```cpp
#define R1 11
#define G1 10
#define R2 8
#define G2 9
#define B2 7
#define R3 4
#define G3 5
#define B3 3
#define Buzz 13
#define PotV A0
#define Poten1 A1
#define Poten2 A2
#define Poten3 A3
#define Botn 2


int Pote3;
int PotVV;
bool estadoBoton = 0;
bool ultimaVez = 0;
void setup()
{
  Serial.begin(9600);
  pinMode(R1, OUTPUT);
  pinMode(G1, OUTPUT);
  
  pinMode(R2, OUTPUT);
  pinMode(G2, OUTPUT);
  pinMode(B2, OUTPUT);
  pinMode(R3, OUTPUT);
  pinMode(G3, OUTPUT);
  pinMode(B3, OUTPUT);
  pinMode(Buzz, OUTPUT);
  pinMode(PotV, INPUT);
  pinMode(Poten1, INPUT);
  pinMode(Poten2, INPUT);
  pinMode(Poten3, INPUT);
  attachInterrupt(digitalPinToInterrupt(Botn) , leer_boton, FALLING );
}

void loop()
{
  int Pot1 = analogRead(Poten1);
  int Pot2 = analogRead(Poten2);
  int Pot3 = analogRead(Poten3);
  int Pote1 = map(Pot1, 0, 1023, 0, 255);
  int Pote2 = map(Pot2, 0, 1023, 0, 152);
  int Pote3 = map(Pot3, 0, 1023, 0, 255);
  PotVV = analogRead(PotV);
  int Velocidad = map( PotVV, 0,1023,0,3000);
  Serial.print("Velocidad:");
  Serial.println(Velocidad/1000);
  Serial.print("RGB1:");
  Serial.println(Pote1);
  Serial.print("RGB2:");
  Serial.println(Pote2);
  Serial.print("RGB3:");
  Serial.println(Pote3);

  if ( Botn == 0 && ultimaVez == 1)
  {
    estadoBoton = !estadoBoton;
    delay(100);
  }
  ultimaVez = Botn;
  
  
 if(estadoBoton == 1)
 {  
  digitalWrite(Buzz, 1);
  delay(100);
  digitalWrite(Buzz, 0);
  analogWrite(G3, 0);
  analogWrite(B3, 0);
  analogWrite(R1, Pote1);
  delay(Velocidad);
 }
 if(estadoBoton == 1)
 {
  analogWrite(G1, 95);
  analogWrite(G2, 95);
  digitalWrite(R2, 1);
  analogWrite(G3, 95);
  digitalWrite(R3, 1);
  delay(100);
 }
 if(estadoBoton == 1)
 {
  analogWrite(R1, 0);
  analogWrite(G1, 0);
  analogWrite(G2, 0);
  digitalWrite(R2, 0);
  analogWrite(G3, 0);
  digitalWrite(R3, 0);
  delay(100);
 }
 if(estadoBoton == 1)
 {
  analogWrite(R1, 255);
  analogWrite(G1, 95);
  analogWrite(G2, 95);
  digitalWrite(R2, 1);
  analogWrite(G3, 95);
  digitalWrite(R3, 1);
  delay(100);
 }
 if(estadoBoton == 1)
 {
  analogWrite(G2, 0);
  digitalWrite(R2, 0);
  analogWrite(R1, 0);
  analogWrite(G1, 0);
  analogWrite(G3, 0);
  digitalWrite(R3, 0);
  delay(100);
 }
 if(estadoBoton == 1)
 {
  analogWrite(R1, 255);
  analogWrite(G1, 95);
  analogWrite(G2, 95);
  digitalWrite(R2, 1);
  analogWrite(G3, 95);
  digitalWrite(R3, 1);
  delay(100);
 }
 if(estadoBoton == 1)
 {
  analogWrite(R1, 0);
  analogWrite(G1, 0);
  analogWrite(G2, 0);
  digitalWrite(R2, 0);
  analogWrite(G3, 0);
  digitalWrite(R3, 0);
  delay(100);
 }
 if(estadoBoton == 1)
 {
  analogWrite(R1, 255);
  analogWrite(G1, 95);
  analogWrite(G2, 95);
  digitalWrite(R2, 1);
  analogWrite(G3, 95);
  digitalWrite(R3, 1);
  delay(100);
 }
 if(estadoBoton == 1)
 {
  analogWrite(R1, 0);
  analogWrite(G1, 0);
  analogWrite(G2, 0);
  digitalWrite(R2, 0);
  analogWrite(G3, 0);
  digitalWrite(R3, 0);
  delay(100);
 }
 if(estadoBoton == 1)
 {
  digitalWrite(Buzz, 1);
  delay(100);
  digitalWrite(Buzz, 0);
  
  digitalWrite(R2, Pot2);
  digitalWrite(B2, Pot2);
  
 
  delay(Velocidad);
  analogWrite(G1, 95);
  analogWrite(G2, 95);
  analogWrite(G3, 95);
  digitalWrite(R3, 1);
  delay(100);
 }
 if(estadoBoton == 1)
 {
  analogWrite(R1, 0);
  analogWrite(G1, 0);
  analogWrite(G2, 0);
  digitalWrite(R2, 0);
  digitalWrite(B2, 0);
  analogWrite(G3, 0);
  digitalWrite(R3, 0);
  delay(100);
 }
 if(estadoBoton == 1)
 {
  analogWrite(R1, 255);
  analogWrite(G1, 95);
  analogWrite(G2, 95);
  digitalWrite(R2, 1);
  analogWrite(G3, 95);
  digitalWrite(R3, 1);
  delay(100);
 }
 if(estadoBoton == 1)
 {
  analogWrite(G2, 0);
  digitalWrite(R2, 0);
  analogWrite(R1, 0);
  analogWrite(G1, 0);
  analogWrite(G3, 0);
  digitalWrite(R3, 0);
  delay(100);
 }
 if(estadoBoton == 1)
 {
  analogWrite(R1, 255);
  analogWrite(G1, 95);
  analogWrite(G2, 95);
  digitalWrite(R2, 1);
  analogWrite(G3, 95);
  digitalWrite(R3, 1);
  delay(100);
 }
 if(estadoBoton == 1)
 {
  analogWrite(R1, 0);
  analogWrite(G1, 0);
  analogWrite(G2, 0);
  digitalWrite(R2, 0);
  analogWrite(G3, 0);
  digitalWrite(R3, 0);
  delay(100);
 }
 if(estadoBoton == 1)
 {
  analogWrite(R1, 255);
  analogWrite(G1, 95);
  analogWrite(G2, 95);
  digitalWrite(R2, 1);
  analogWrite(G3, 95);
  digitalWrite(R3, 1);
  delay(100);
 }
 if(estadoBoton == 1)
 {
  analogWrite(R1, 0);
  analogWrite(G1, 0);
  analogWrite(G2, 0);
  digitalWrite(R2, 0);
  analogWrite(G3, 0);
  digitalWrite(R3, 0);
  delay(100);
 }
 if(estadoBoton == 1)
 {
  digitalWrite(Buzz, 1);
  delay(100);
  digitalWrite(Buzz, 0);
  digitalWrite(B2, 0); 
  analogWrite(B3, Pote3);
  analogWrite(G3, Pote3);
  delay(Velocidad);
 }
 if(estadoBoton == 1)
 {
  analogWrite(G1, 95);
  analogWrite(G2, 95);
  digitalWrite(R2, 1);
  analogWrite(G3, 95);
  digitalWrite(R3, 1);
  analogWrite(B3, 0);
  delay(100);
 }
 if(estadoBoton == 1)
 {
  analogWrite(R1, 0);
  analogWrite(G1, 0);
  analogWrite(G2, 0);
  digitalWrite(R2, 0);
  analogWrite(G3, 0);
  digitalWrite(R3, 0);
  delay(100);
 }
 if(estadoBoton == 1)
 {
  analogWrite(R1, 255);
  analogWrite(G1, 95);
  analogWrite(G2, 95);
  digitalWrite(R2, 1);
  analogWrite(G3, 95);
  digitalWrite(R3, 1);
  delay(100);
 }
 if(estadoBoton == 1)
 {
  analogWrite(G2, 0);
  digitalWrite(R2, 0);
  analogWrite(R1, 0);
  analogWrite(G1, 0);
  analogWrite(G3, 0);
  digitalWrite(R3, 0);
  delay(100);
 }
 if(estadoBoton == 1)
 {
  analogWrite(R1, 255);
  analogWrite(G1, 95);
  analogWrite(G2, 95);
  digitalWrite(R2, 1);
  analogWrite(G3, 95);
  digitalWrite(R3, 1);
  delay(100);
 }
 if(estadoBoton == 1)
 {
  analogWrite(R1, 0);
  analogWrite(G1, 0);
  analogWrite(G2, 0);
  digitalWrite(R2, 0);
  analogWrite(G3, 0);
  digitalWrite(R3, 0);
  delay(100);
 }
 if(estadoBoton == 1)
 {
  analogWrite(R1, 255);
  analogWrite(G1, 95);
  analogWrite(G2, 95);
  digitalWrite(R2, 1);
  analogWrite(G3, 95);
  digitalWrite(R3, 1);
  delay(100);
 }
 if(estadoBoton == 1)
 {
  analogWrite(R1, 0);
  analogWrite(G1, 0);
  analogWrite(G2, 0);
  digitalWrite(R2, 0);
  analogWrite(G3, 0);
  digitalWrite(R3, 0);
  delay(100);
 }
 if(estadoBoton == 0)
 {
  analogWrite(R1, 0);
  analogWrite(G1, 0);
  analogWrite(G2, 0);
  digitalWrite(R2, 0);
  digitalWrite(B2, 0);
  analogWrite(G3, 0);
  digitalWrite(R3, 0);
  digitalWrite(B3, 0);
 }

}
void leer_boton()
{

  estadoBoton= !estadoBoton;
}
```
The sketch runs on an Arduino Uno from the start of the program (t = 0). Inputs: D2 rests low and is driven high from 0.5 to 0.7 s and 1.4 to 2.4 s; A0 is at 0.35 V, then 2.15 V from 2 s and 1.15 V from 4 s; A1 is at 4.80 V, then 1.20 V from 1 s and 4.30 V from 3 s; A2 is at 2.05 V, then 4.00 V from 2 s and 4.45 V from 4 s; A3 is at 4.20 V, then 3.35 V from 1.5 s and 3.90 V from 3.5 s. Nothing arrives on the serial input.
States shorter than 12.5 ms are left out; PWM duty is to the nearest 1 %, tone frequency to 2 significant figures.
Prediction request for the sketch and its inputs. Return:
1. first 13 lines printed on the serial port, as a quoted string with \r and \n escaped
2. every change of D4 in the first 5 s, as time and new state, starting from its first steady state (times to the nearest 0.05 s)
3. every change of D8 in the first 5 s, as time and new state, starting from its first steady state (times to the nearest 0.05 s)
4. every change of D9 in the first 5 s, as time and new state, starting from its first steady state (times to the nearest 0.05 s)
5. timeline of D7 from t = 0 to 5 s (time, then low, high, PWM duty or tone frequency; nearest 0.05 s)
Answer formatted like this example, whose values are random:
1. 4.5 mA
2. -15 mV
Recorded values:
1. "Velocidad:0\r\nRGB1:245\r\nRGB2:62\r\nRGB3:214\r\nVelocidad:0\r\nRGB1:245\r\nRGB2:62\r\nRGB3:214\r\nVelocidad:0\r\nRGB1:245\r\nRGB2:62\r\nRGB3:214\r\nVelocidad:0\r\n"
2. 0 s low; 1.05 s high; 1.15 s low; 1.25 s high; 1.35 s low; 1.45 s high; 1.55 s low; 1.65 s high; 1.75 s low; 2.15 s high; 2.25 s low; 2.35 s high; 2.45 s low
3. 0 s low; 1.05 s high; 1.15 s low; 1.25 s high; 1.35 s low; 1.45 s high; 1.55 s low; 1.65 s high; 1.75 s low; 1.95 s high; 2.25 s low; 2.35 s high; 2.45 s low
4. 0 s low; 1.05 s PWM 37 %; 1.15 s low; 1.25 s PWM 37 %; 1.35 s low; 1.45 s PWM 37 %; 1.55 s low; 1.65 s PWM 37 %; 1.75 s low; 2.15 s PWM 37 %; 2.25 s low; 2.35 s PWM 37 %; 2.45 s low
5. 0 s low; 1.95 s high; 2.25 s low
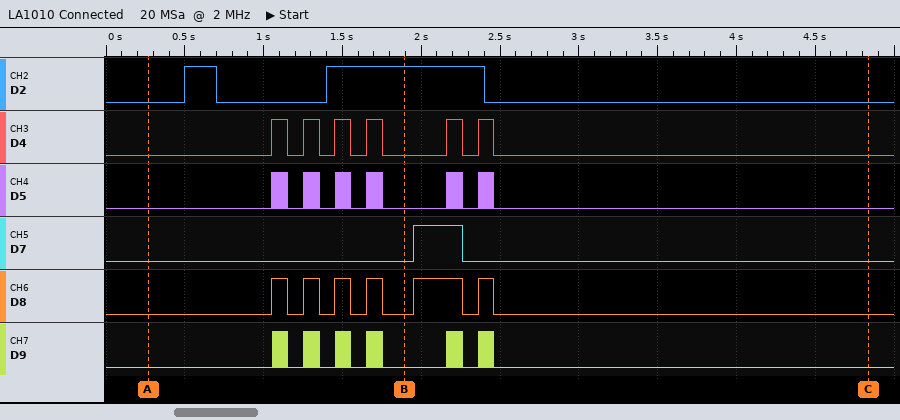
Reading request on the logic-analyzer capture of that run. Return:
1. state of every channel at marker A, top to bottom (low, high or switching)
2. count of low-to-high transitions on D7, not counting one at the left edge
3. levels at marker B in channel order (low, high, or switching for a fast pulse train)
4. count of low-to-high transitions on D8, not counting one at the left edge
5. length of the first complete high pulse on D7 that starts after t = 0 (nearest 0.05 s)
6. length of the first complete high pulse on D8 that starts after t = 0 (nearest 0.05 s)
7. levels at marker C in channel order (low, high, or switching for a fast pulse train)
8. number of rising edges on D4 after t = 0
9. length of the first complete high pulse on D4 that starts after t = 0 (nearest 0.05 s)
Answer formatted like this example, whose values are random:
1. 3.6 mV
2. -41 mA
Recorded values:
1. D2 low, D4 low, D5 low, D7 low, D8 low, D9 low
2. 1
3. D2 high, D4 low, D5 low, D7 low, D8 low, D9 low
4. 6
5. 0.30 s
6. 0.10 s
7. D2 low, D4 low, D5 low, D7 low, D8 low, D9 low
8. 6
9. 0.10 s
